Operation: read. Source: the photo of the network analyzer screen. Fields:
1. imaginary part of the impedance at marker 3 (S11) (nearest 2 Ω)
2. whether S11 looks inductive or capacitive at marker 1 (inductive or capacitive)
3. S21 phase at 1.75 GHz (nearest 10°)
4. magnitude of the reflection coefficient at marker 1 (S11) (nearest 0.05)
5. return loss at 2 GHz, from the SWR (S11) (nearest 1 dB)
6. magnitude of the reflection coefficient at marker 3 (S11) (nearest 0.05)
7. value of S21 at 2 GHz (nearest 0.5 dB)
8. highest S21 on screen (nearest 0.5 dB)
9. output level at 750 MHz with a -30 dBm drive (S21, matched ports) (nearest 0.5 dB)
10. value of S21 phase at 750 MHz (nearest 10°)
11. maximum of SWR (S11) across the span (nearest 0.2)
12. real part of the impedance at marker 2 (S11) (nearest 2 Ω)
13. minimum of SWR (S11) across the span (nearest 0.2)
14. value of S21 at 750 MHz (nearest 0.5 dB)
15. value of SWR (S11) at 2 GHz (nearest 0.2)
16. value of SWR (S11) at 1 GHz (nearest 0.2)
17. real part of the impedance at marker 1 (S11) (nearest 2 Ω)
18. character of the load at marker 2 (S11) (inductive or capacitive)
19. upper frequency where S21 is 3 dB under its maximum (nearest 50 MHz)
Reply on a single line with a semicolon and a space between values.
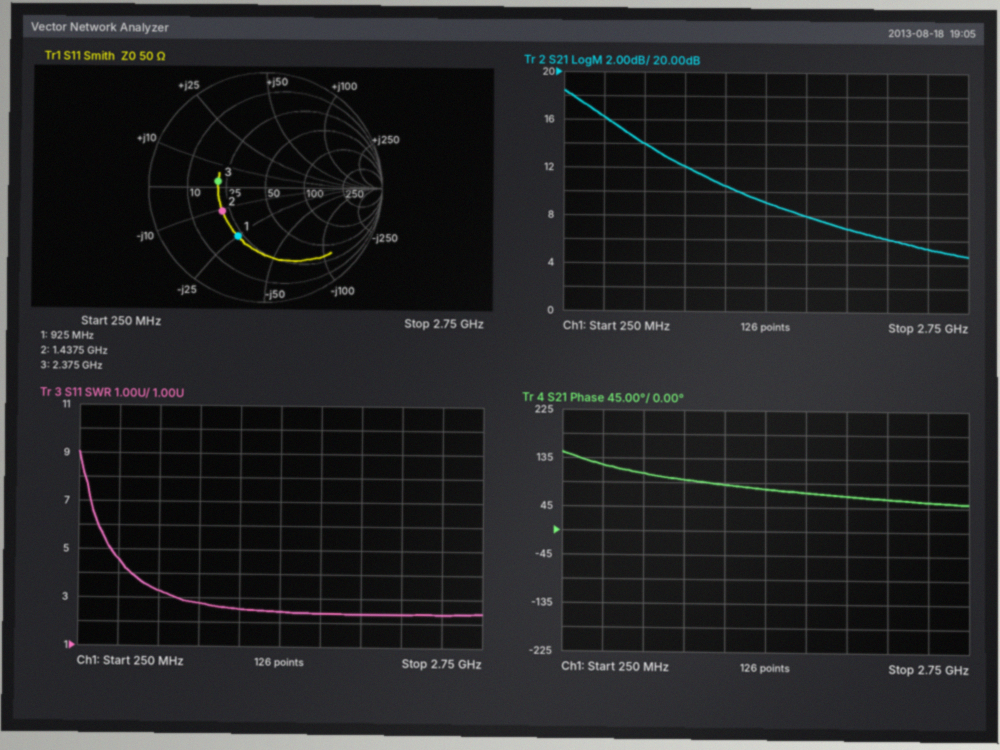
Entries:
+2 Ω; capacitive; 70°; 0.50; 8 dB; 0.40; 7.0 dB; 18.5 dB; -16.0 dBm; 110°; 9.0; 22 Ω; 2.4; 14.0 dB; 2.4; 2.8; 22 Ω; capacitive; 600 MHz
